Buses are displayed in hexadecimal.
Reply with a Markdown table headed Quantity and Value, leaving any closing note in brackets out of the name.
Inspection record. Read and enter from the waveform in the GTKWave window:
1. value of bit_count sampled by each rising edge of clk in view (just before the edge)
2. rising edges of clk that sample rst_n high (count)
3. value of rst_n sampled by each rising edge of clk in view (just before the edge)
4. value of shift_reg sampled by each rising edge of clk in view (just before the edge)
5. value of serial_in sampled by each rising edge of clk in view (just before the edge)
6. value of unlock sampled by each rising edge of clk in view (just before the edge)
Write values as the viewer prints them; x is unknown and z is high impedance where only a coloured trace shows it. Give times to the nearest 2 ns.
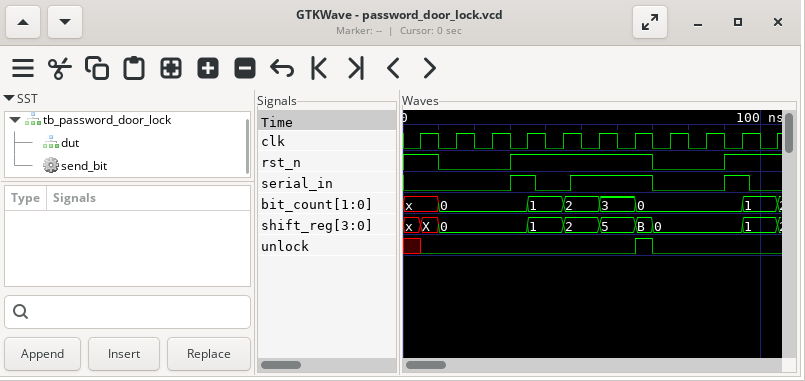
| Quantity | Value |
|---|---|
| value of bit_count sampled by each rising edge of clk in view | x, 0, 0, 0, 1, 2, 3, 0, 0, 0, 1 |
| rising edges of clk that sample rst_n high | 7 |
| value of rst_n sampled by each rising edge of clk in view | 1 0 0 1 1 1 1 0 0 1 1 |
| value of shift_reg sampled by each rising edge of clk in view | x, 0, 0, 0, 1, 2, 5, 0, 0, 0, 1 |
| value of serial_in sampled by each rising edge of clk in view | 0 0 0 1 0 1 1 0 0 1 0 |
| value of unlock sampled by each rising edge of clk in view | x 0 0 0 0 0 0 0 0 0 0 |
